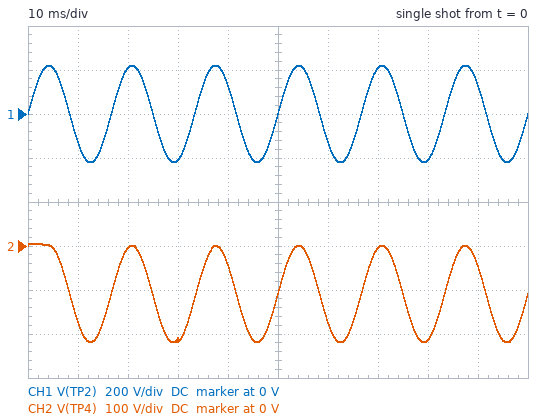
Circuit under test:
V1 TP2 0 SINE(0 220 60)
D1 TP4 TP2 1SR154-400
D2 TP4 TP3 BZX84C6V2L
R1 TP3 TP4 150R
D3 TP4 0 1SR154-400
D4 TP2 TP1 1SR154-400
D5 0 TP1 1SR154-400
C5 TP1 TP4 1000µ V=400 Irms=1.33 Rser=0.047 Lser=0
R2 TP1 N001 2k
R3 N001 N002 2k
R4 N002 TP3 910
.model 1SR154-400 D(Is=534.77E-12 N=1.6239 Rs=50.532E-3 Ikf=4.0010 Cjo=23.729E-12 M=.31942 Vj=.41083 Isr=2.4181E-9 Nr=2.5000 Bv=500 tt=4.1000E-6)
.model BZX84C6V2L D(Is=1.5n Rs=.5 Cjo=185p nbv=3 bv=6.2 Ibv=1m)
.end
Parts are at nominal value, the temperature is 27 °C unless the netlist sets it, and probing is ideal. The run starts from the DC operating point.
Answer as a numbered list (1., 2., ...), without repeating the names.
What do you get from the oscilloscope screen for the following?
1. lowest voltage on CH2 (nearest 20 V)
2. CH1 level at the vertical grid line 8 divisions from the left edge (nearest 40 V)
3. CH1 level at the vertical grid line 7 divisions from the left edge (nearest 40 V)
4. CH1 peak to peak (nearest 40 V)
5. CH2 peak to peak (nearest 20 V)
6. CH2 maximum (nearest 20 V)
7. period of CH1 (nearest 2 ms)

1. -220 V
2. -200 V
3. 200 V
4. 440 V
5. 220 V
6. 0 V
7. 16 ms
